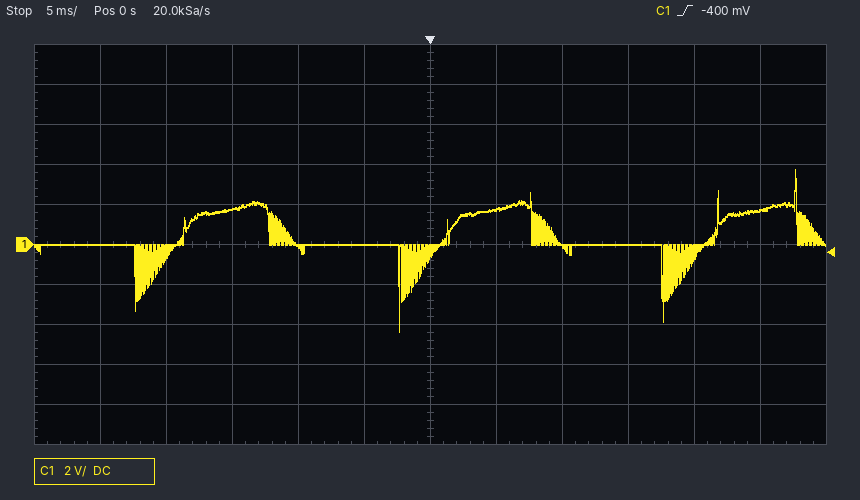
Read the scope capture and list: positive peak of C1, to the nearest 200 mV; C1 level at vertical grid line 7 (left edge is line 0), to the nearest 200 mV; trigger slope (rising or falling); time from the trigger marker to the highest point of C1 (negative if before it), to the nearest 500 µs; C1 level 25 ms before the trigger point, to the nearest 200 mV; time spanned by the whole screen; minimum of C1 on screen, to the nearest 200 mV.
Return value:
3.8 V
1.8 V
rising
+27.5 ms
0.0 V
60 ms
-4.4 V
